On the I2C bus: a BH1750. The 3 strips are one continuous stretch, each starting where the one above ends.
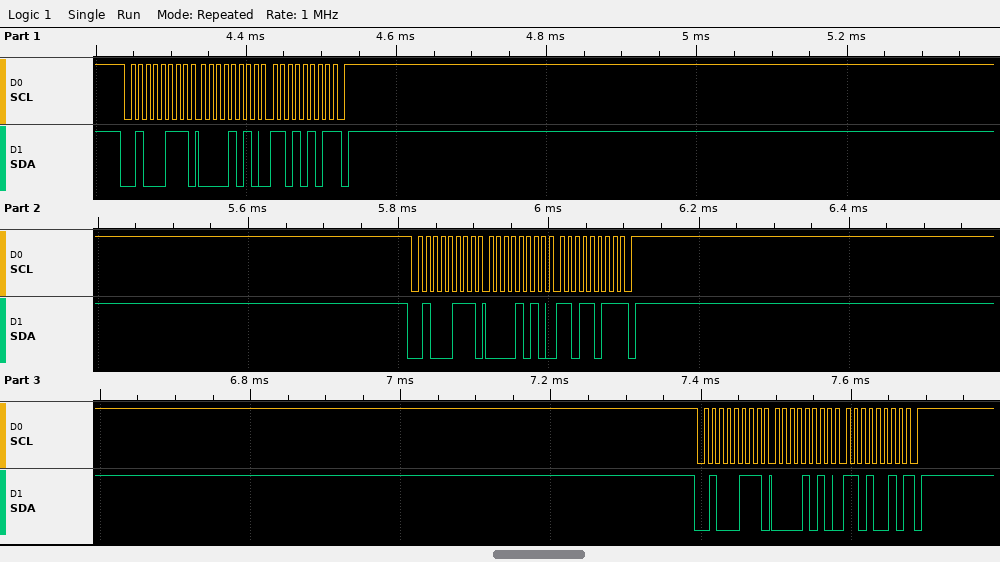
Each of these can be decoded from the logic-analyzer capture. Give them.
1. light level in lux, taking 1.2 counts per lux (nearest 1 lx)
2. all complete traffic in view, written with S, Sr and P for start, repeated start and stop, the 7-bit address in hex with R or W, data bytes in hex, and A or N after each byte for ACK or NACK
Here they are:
2311 lx
S 23R A 0A A D5 N P S 23R A 0A A DB N P S 23R A 0A A D2 N P
